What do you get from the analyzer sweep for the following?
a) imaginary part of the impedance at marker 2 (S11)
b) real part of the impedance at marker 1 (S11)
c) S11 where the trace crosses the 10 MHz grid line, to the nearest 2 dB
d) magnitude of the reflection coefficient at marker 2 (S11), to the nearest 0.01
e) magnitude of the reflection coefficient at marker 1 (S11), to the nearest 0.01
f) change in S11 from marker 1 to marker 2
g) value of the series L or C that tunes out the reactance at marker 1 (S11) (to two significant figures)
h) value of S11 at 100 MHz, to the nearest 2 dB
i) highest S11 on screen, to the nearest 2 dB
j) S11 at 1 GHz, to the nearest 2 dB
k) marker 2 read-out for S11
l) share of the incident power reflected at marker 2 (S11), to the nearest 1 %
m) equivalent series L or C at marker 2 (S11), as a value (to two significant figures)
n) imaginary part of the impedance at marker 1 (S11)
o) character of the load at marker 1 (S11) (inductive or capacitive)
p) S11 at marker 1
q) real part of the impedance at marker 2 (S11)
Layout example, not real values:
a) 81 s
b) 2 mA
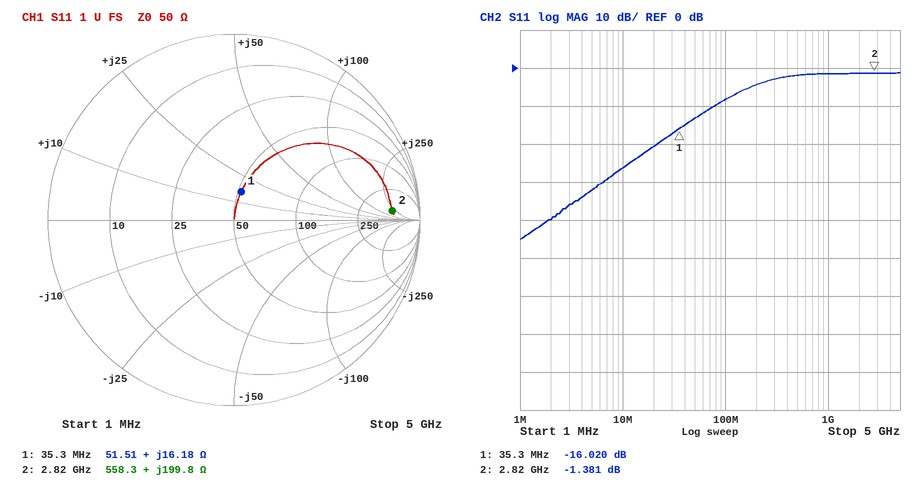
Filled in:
a) +199.8 Ω
b) 51.51 Ω
c) -26 dB
d) 0.85
e) 0.16
f) 14.639 dB
g) 280 pF
h) -8 dB
i) -2 dB
j) -2 dB
k) -1.381 dB
l) 73 %
m) 11 nH
n) +16.18 Ω
o) inductive
p) -16.020 dB
q) 558.3 Ω
